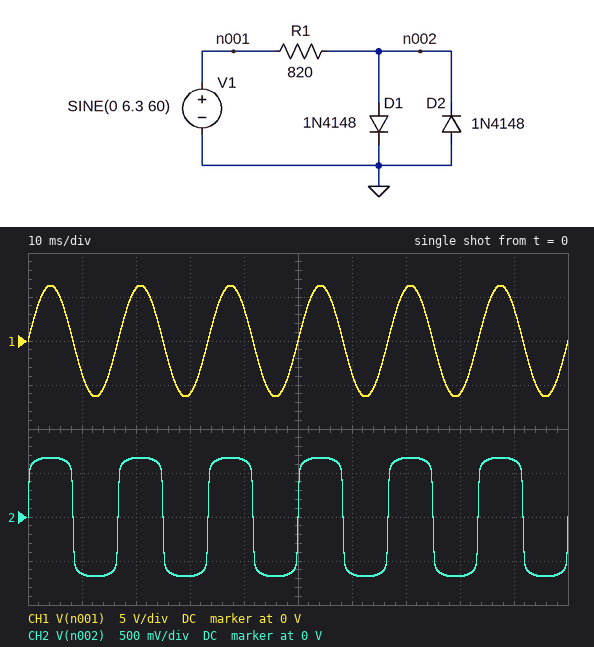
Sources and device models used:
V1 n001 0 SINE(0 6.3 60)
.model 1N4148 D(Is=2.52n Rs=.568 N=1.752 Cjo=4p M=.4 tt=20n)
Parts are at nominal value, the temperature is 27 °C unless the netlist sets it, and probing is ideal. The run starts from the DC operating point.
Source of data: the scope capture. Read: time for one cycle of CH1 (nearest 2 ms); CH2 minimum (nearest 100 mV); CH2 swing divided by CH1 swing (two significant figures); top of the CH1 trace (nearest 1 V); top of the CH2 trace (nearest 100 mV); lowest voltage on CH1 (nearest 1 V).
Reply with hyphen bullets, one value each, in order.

- 16 ms
- -700 mV
- 0.11
- 6 V
- 700 mV
- -6 V
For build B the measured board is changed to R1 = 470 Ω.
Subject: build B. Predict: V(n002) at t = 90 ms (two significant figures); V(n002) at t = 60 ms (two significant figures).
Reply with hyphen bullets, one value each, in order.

- 670 mV
- -670 mV
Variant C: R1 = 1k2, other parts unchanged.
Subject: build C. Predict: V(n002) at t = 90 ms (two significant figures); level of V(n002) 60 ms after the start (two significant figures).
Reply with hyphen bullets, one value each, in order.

- 630 mV
- -630 mV
